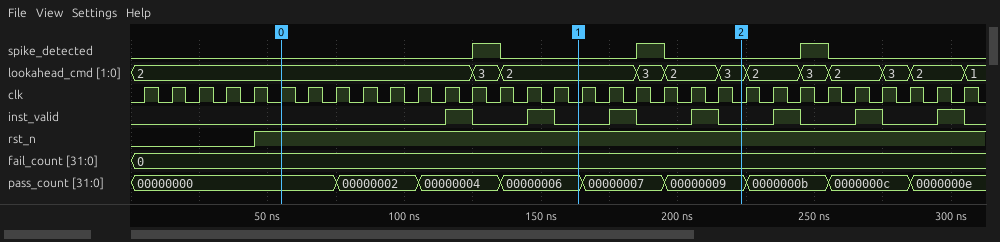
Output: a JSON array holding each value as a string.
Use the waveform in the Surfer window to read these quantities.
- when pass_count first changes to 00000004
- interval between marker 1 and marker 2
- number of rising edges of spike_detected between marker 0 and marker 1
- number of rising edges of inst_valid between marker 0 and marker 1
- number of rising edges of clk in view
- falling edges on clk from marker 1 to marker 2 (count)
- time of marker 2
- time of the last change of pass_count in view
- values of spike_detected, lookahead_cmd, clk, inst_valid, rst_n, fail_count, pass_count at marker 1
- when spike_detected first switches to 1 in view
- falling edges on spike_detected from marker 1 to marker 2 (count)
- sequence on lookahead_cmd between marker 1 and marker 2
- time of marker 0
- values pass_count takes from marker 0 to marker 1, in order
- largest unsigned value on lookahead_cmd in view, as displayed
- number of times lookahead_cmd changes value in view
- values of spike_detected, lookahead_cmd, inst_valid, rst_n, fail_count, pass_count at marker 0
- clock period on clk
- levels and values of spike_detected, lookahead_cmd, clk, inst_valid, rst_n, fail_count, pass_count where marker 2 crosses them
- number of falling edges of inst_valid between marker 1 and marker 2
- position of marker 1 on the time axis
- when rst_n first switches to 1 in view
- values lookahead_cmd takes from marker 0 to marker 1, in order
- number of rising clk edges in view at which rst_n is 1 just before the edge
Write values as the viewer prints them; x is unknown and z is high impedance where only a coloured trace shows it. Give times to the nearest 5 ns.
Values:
["105 ns", "60 ns", "1", "2", "31", "6", "225 ns", "285 ns", "spike_detected=0, lookahead_cmd=2, clk=0, inst_valid=0, rst_n=1, fail_count=0, pass_count=00000006", "125 ns", "1", "2, 3, 2, 3", "55 ns", "00000000, 00000002, 00000004, 00000006", "3", "11", "spike_detected=0, lookahead_cmd=2, inst_valid=0, rst_n=1, fail_count=0, pass_count=00000000", "10 ns", "spike_detected=0, lookahead_cmd=3, clk=0, inst_valid=0, rst_n=1, fail_count=0, pass_count=00000009", "2", "165 ns", "45 ns", "2, 3, 2", "26"]
